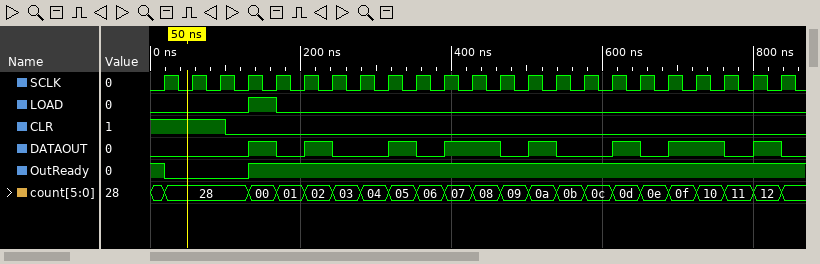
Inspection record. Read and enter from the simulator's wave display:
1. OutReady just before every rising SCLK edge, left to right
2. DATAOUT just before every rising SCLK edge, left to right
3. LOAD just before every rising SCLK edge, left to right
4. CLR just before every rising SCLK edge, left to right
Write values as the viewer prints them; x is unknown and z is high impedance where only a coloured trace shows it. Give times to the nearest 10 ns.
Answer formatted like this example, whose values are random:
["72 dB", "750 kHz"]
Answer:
["1 0 0 0 1 1 1 1 1 1 1 1 1 1 1 1 1 1 1 1 1 1 1", "0 0 0 0 1 0 1 0 0 1 0 1 1 0 1 0 0 1 0 1 1 0 1", "0 0 0 0 1 0 0 0 0 0 0 0 0 0 0 0 0 0 0 0 0 0 0", "1 1 1 0 0 0 0 0 0 0 0 0 0 0 0 0 0 0 0 0 0 0 0"]
